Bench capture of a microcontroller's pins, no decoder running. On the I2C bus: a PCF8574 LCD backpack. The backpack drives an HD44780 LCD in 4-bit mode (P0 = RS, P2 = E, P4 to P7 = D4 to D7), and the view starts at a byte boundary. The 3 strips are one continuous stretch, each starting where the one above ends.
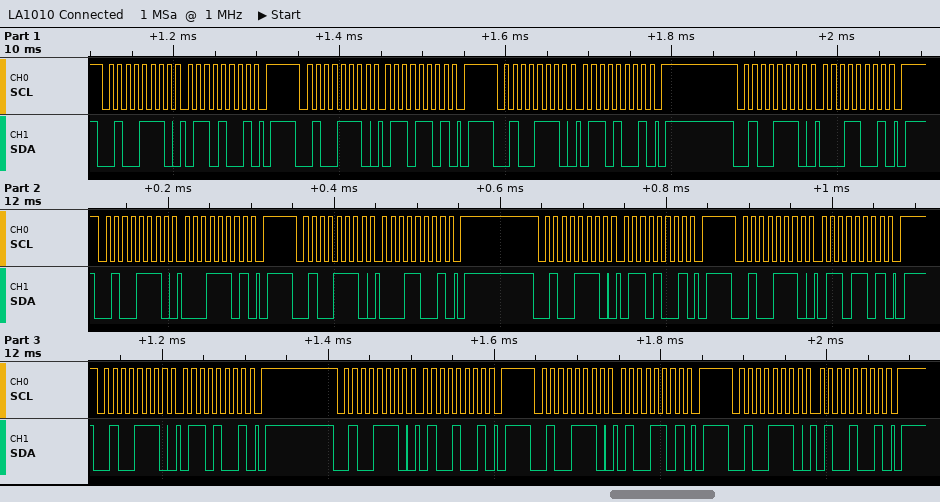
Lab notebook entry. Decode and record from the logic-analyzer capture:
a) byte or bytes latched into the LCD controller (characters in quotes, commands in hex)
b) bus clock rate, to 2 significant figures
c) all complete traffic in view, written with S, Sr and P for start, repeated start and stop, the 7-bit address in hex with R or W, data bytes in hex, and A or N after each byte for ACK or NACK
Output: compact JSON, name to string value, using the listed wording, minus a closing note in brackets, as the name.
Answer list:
{"byte or bytes latched into the LCD controller": "'a' 'd'", "bus clock rate, to 2 significant figures": "100 kHz", "all complete traffic in view, written with S, Sr and P for start, repeated start and stop, the 7-bit address in hex with R or W, data bytes in hex, and A or N after each byte for ACK or NACK": "S 27W A 69 A P S 27W A 6D A P S 27W A 69 A P S 27W A 19 A P S 27W A 1D A P S 27W A 19 A P S 27W A 69 A P S 27W A 6D A P S 27W A 69 A P S 27W A 49 A P S 27W A 4D A P S 27W A 49 A P"}
